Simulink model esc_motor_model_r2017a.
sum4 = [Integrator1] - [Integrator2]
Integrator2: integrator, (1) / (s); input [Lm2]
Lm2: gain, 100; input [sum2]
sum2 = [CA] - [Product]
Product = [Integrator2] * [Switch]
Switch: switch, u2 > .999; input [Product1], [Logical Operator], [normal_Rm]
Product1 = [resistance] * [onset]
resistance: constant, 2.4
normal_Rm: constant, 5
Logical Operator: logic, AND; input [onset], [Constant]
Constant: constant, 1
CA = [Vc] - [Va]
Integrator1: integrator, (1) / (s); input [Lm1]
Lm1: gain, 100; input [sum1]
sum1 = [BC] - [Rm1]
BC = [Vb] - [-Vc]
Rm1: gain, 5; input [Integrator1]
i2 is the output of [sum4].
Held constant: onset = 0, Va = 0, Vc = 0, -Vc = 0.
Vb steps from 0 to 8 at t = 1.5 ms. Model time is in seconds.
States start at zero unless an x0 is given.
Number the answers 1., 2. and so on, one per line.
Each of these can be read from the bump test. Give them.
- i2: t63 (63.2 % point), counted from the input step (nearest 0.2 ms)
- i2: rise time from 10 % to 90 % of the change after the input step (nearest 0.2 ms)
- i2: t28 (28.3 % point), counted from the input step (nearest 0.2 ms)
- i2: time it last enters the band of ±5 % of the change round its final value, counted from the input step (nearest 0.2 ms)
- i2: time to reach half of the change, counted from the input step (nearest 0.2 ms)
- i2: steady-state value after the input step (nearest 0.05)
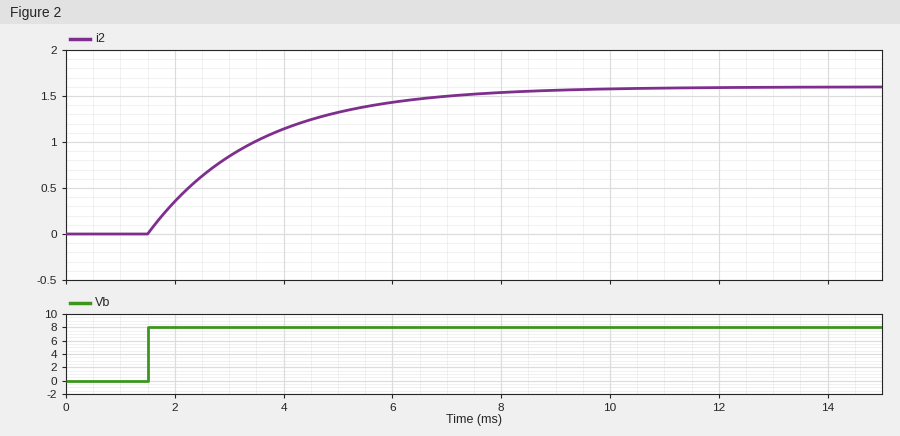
1. 2.0 ms
2. 4.4 ms
3. 0.6 ms
4. 6.0 ms
5. 1.4 ms
6. 1.60
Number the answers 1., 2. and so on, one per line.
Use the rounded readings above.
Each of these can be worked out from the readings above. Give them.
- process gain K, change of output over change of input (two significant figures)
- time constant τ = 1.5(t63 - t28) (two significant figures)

1. 0.20
2. 2.1 ms
